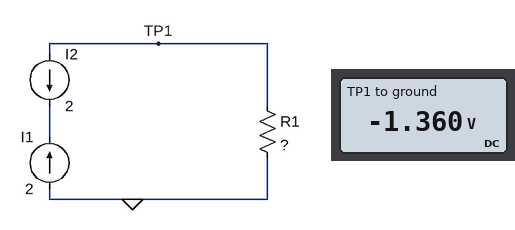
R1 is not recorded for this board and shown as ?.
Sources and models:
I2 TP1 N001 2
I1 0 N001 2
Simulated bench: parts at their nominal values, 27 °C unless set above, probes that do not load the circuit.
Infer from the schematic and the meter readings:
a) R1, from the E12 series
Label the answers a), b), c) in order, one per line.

a) 0.68 Ω
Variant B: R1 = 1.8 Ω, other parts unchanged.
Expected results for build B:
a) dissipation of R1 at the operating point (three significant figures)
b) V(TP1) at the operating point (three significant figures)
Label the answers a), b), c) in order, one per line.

a) 7.20 W
b) -3.60 V
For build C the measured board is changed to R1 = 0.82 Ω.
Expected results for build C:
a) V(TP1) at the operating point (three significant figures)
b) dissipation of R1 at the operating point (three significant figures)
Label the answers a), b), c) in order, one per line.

a) -1.64 V
b) 3.28 W
